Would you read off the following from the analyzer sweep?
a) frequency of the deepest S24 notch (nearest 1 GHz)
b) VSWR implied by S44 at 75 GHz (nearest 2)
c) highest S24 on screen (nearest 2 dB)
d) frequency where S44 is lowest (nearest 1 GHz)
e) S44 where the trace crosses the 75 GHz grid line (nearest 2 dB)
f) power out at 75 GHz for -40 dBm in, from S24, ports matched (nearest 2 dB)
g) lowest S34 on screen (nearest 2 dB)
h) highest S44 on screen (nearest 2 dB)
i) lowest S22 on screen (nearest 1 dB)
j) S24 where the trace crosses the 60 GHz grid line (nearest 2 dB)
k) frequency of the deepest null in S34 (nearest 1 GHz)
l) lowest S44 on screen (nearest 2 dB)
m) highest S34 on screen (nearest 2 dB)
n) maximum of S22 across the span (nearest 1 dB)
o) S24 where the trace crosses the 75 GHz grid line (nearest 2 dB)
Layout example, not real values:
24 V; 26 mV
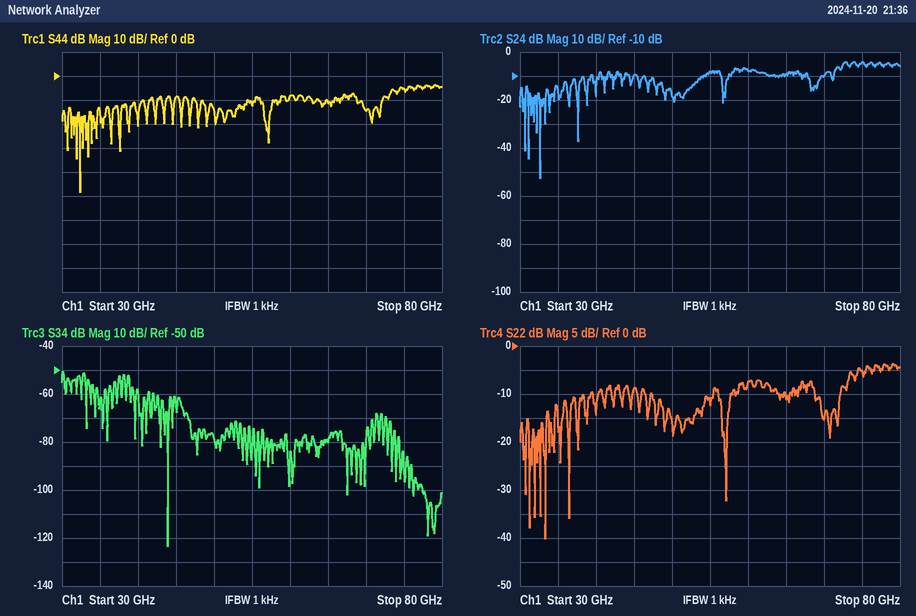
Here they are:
33 GHz; 4; -4 dB; 32 GHz; -6 dB; -44 dBm; -124 dB; -4 dB; -40 dB; -8 dB; 44 GHz; -48 dB; -50 dB; -4 dB; -4 dB
